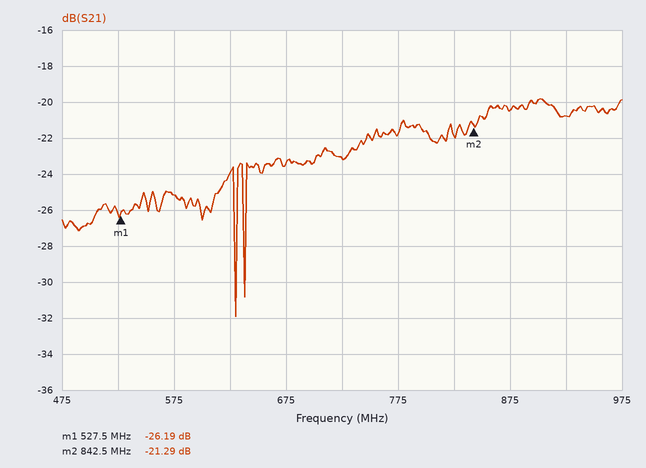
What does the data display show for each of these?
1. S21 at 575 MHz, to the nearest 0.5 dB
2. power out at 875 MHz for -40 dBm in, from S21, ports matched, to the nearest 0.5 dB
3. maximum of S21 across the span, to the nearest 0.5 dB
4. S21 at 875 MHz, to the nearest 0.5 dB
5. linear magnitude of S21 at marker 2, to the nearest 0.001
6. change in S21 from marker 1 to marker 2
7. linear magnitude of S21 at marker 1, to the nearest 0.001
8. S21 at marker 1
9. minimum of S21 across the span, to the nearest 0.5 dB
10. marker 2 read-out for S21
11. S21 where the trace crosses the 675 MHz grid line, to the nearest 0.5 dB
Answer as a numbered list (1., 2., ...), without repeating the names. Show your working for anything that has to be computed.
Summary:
1. -25.0 dB
2. -40 dBm + (-20.5 dB) = -60.5 dBm
3. -20.0 dB
4. -20.5 dB
5. 10^(-21.29/20) ≈ 0.086
6. -21.29 − (-26.19) = 4.90 dB
7. 10^(-26.19/20) ≈ 0.049
8. -26.19 dB
9. -32.0 dB
10. -21.29 dB
11. -23.5 dB
